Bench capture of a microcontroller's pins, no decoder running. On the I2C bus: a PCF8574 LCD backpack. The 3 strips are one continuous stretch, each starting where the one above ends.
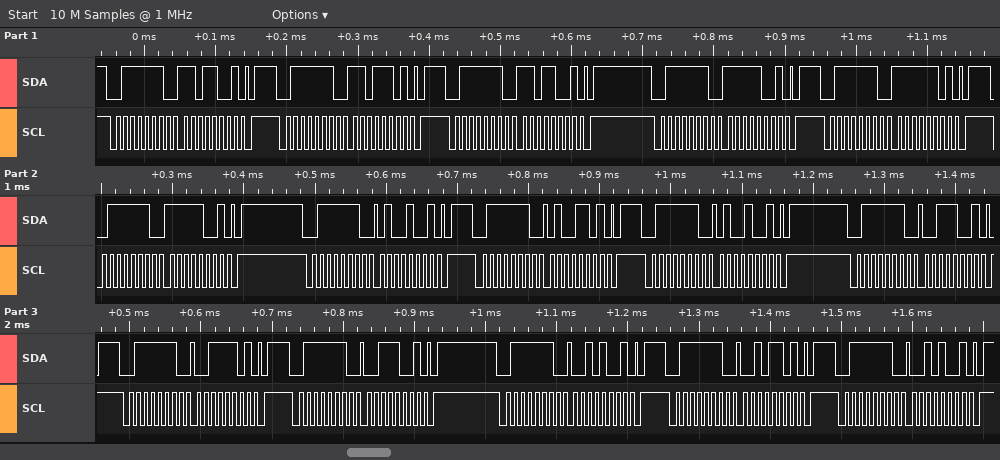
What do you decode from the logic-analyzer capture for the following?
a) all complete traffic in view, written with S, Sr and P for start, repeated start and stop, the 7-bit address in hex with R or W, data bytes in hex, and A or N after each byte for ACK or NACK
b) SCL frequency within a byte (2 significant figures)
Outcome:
S 3FW A D9 A P S 3FW A DD A P S 3FW A D9 A P S 3FW A F9 A P S 3FW A FD A P S 3FW A F9 A P S 3FW A 49 A P S 3FW A 4D A P S 3FW A 49 A P S 3FW A 39 A P S 3FW A 3D A P S 3FW A 39 A P S 3FW A 29 A P S 3FW A 2D A P S 3FW A 29 A P
100 kHz
